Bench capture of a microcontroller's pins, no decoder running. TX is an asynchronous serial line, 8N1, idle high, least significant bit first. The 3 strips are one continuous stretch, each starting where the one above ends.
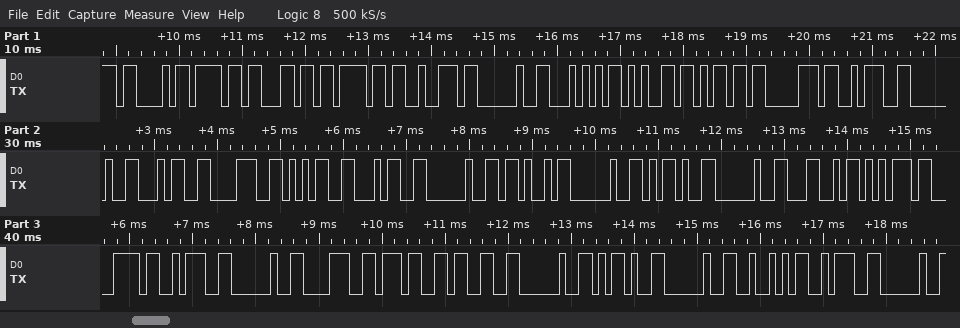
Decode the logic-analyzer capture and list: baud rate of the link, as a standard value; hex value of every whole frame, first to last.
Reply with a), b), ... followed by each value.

a) 9600 baud
b) 43 6F 6C 6F 72 20 54 65 6D 70 3A 20 34 38 35 34 20 4B 20 2D 20 4C 75 78 3A 20 38 37 33 20 2D 20 52 3A 20
